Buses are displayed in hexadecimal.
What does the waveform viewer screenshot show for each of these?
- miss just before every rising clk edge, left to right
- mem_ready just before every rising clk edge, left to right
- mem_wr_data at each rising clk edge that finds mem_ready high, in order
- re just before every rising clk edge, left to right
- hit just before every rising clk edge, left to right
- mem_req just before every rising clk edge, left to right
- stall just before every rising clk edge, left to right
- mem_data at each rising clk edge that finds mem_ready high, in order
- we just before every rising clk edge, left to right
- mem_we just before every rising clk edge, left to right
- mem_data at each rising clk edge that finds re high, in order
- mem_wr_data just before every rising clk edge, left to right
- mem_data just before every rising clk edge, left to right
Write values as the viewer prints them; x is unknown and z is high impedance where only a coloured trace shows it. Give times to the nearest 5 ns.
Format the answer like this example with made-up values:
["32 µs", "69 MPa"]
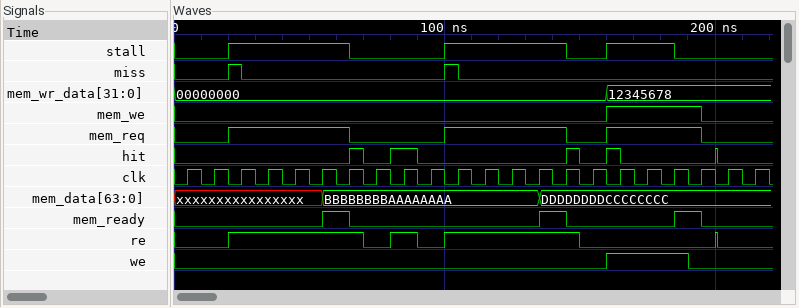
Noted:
["0 0 1 0 0 0 0 0 0 0 1 0 0 0 0 0 0 0 0 0 0 0", "0 0 0 0 0 0 1 0 0 0 0 0 0 0 1 0 0 0 0 1 0 0", "00000000, 00000000, 12345678", "0 0 1 1 1 1 1 0 1 0 1 1 1 1 1 0 0 0 0 0 0 0", "0 0 0 0 0 0 0 0 1 0 0 0 0 0 0 0 1 0 0 0 0 0", "0 0 1 1 1 1 1 0 0 0 1 1 1 1 1 0 1 1 1 1 0 0", "0 0 1 1 1 1 1 0 0 0 1 1 1 1 1 0 1 1 1 0 0 0", "BBBBBBBBAAAAAAAA, DDDDDDDDCCCCCCCC, DDDDDDDDCCCCCCCC", "0 0 0 0 0 0 0 0 0 0 0 0 0 0 0 0 1 1 1 0 0 0", "0 0 0 0 0 0 0 0 0 0 0 0 0 0 0 0 1 1 1 1 0 0", "xxxxxxxxxxxxxxxx, xxxxxxxxxxxxxxxx, xxxxxxxxxxxxxxxx, xxxxxxxxxxxxxxxx, BBBBBBBBAAAAAAAA, BBBBBBBBAAAAAAAA, BBBBBBBBAAAAAAAA, BBBBBBBBAAAAAAAA, BBBBBBBBAAAAAAAA, BBBBBBBBAAAAAAAA, DDDDDDDDCCCCCCCC", "00000000, 00000000, 00000000, 00000000, 00000000, 00000000, 00000000, 00000000, 00000000, 00000000, 00000000, 00000000, 00000000, 00000000, 00000000, 00000000, 12345678, 12345678, 12345678, 12345678, 12345678, 12345678", "xxxxxxxxxxxxxxxx, xxxxxxxxxxxxxxxx, xxxxxxxxxxxxxxxx, xxxxxxxxxxxxxxxx, xxxxxxxxxxxxxxxx, xxxxxxxxxxxxxxxx, BBBBBBBBAAAAAAAA, BBBBBBBBAAAAAAAA, BBBBBBBBAAAAAAAA, BBBBBBBBAAAAAAAA, BBBBBBBBAAAAAAAA, BBBBBBBBAAAAAAAA, BBBBBBBBAAAAAAAA, BBBBBBBBAAAAAAAA, DDDDDDDDCCCCCCCC, DDDDDDDDCCCCCCCC, DDDDDDDDCCCCCCCC, DDDDDDDDCCCCCCCC, DDDDDDDDCCCCCCCC, DDDDDDDDCCCCCCCC, DDDDDDDDCCCCCCCC, DDDDDDDDCCCCCCCC"]
